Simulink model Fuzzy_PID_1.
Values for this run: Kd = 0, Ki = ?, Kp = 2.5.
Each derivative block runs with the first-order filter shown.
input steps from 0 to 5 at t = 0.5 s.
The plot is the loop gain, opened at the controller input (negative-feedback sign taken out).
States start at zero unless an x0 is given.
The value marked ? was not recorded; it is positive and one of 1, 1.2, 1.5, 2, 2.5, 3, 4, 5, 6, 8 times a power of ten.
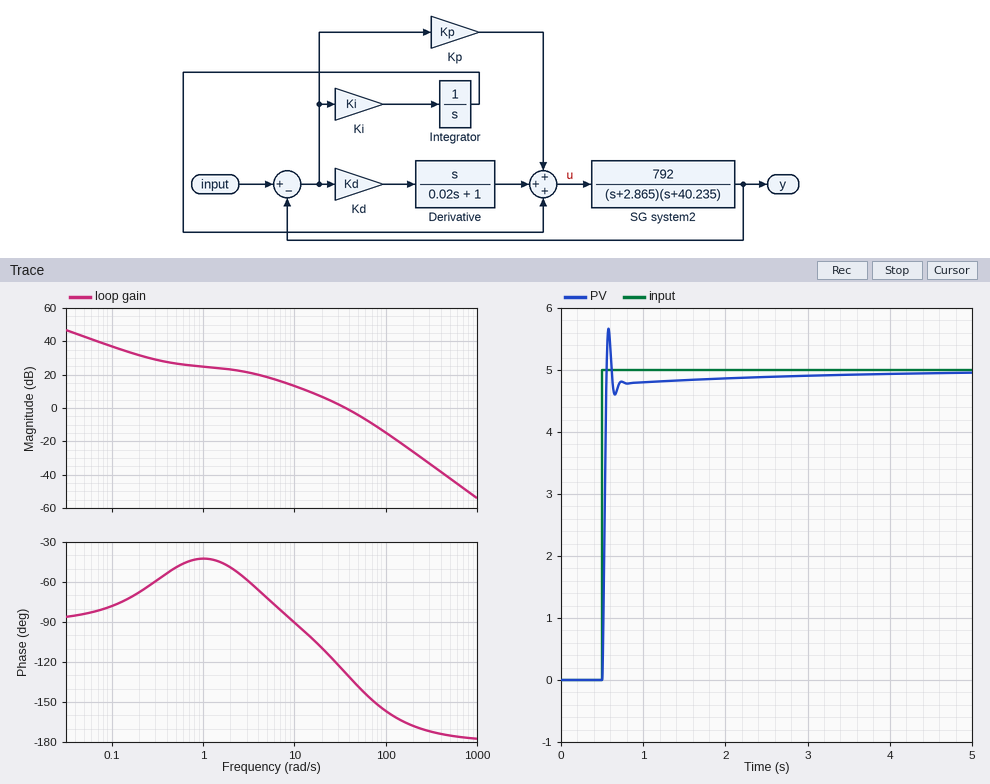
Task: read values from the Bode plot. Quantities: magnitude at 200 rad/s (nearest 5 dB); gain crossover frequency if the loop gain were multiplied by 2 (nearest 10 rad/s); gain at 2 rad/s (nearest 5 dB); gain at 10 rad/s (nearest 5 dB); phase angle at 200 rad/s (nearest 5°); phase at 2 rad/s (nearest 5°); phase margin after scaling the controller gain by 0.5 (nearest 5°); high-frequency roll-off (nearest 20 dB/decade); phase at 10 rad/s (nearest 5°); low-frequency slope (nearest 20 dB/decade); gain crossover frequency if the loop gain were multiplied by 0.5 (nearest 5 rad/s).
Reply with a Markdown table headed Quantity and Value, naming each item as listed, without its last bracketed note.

| Quantity | Value |
|---|---|
| magnitude at 200 rad/s | -25 dB |
| gain crossover frequency if the loop gain were multiplied by 2 | 60 rad/s |
| gain at 2 rad/s | 25 dB |
| gain at 10 rad/s | 15 dB |
| phase angle at 200 rad/s | -170° |
| phase at 2 rad/s | -50° |
| phase margin after scaling the controller gain by 0.5 | 70° |
| high-frequency roll-off | -40 dB/decade |
| phase at 10 rad/s | -90° |
| low-frequency slope | -20 dB/decade |
| gain crossover frequency if the loop gain were multiplied by 0.5 | 20 rad/s |
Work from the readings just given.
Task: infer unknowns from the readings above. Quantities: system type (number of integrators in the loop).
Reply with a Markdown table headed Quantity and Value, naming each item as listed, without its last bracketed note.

| Quantity | Value |
|---|---|
| system type | 1 |
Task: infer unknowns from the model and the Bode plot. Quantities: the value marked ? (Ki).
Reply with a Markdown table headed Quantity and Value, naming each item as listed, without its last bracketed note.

| Quantity | Value |
|---|---|
| the value marked ? | 1 |
